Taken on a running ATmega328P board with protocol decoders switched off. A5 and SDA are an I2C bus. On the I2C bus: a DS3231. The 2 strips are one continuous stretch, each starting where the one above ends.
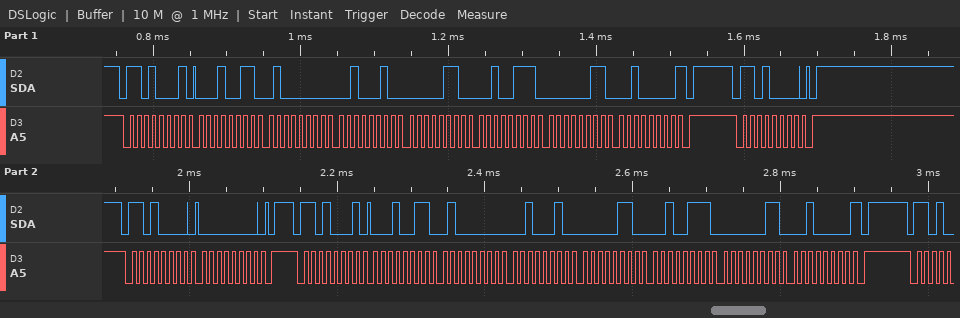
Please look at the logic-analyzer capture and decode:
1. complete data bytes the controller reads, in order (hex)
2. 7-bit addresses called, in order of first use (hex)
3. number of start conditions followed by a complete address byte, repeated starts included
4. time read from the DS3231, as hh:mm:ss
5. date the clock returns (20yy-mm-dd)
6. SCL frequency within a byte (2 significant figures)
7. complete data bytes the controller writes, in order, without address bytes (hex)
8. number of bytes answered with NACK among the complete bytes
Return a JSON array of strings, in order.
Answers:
["13 40 22 06 27 03 20 13 40 22 06 27 03 20", "0x68", "4", "22:40:13", "2020-03-27", "100 kHz", "00", "2"]
